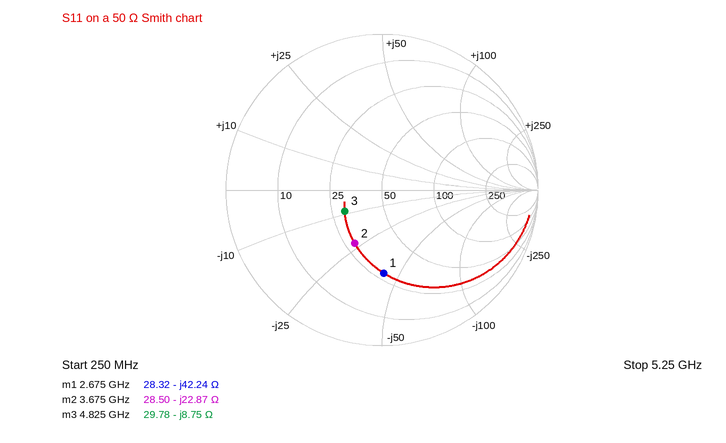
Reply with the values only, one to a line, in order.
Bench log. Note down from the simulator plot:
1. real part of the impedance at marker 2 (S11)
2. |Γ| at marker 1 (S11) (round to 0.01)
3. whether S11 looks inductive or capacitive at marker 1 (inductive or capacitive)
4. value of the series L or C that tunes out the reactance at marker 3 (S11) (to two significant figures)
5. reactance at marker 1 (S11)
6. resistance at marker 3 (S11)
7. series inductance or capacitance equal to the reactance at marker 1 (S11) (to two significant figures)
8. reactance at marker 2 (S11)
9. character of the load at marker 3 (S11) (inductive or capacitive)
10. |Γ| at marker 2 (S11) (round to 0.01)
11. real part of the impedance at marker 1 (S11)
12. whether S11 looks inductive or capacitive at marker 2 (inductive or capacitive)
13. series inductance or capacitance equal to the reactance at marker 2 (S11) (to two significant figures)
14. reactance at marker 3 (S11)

28.50 Ω
0.53
capacitive
290 pH
-42.24 Ω
29.78 Ω
1.4 pF
-22.87 Ω
capacitive
0.38
28.32 Ω
capacitive
1.9 pF
-8.75 Ω
